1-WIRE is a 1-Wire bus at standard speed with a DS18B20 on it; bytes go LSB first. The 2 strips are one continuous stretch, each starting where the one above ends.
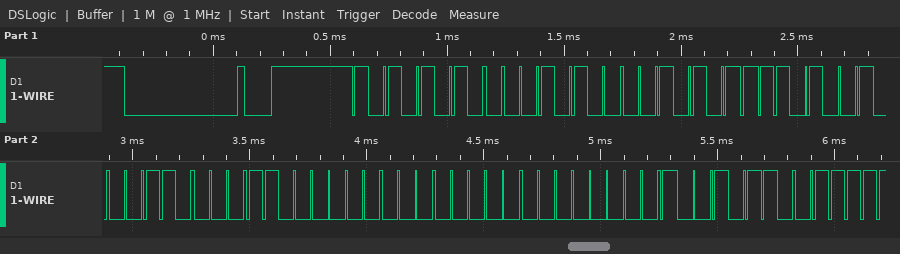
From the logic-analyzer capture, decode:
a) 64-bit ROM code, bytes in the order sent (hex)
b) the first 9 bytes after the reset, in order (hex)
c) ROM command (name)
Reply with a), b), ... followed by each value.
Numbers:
a) 28 D4 4B 0C 03 00 00 69
b) 55 28 D4 4B 0C 03 00 00 69
c) Match ROM
